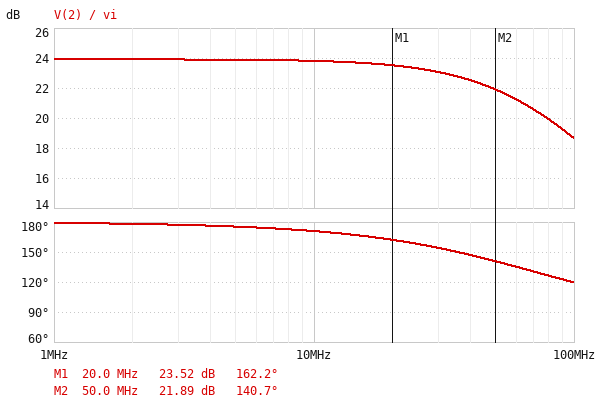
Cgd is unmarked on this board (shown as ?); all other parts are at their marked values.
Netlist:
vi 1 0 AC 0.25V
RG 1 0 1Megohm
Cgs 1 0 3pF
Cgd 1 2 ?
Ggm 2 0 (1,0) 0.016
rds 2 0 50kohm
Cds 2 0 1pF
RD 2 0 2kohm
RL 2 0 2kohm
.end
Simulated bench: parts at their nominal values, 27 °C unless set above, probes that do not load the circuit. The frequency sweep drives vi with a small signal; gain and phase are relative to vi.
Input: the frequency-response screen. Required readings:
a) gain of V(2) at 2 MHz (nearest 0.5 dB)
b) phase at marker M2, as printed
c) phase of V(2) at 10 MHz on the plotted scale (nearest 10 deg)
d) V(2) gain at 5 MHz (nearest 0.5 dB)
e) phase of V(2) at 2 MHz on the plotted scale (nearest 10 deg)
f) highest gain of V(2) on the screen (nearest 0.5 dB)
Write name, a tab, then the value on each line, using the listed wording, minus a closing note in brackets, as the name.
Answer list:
gain of V(2) at 2 MHz	24.0 dB
phase at marker M2, as printed	140.7 deg
phase of V(2) at 10 MHz on the plotted scale	170 deg
V(2) gain at 5 MHz	24.0 dB
phase of V(2) at 2 MHz on the plotted scale	180 deg
highest gain of V(2) on the screen	24.0 dB
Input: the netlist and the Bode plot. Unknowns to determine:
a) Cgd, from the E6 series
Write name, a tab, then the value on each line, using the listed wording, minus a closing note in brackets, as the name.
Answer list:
Cgd, from the E6 series	1.5 pF
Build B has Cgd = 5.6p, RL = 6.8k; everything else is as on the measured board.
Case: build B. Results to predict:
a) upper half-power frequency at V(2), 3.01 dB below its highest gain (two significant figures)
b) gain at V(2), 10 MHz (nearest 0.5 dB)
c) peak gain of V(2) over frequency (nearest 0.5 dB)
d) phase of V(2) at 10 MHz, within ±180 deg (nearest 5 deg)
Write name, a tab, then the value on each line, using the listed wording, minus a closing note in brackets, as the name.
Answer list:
upper half-power frequency at V(2), 3.01 dB below its highest gain	16 MHz
gain at V(2), 10 MHz	26.0 dB
peak gain of V(2) over frequency	27.5 dB
phase of V(2) at 10 MHz, within ±180 deg	145 deg
